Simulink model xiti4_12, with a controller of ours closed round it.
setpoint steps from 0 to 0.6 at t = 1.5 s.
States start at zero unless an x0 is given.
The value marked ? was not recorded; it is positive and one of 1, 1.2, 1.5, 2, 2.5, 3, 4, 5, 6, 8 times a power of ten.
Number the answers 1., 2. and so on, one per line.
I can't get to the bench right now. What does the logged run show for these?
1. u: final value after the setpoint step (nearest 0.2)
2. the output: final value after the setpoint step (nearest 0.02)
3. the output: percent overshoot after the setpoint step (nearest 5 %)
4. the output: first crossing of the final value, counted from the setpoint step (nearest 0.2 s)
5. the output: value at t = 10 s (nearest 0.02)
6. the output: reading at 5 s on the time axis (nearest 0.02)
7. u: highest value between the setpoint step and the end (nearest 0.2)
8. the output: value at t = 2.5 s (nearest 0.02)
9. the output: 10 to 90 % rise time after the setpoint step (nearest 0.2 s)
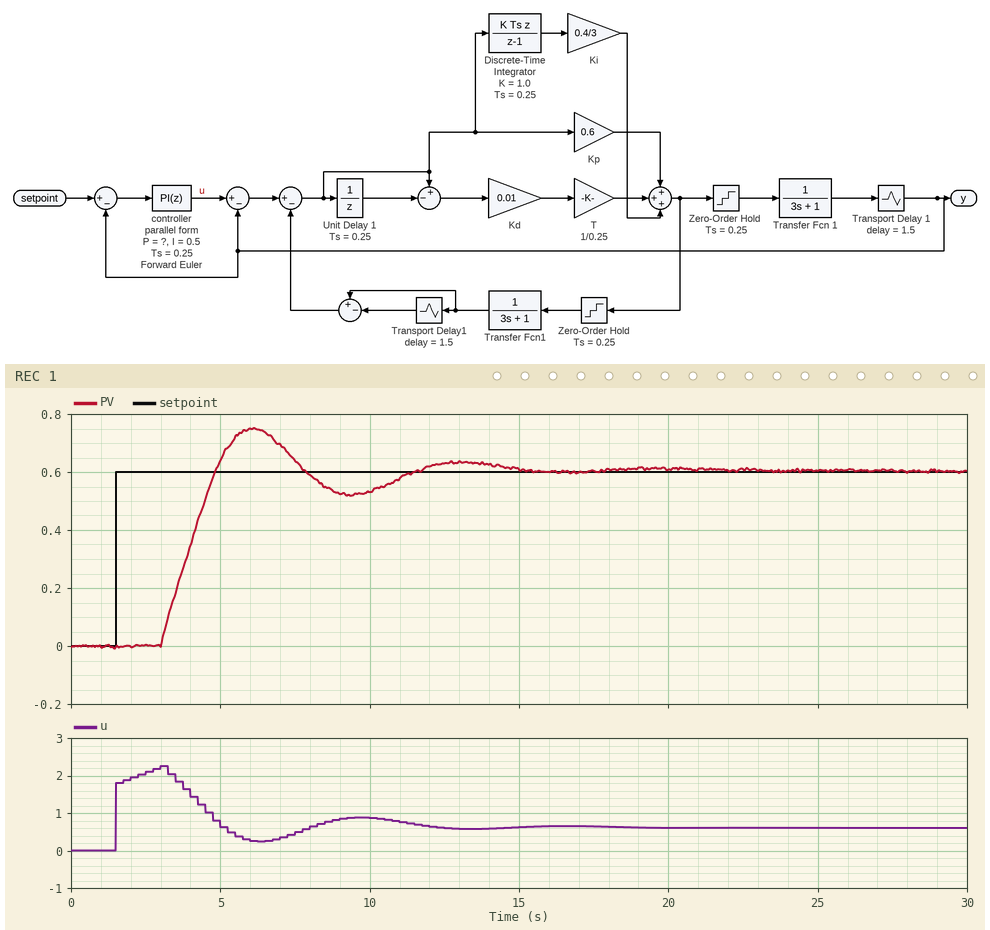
1. 0.6
2. 0.60
3. 25 %
4. 3.4 s
5. 0.54
6. 0.64
7. 2.2
8. 0.00
9. 1.4 s
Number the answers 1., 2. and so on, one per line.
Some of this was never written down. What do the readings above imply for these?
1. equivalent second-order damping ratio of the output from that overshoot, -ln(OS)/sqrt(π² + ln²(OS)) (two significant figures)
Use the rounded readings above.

1. 0.40
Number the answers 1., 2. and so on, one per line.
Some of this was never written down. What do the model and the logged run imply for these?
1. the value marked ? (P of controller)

1. 3
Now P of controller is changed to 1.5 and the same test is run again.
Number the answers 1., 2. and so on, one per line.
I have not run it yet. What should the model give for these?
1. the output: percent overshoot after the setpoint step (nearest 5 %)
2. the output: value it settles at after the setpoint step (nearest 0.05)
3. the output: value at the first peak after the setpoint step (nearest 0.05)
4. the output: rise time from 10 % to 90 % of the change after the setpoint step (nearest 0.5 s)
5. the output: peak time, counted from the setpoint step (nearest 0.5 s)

1. 15 %
2. 0.60
3. 0.70
4. 3.0 s
5. 8.5 s
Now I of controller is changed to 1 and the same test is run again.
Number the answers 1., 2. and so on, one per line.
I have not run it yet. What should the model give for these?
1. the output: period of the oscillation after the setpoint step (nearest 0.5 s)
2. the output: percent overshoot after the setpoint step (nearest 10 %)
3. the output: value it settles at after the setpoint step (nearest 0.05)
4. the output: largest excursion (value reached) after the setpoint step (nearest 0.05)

1. 8.0 s
2. 60 %
3. 0.60
4. 0.95
